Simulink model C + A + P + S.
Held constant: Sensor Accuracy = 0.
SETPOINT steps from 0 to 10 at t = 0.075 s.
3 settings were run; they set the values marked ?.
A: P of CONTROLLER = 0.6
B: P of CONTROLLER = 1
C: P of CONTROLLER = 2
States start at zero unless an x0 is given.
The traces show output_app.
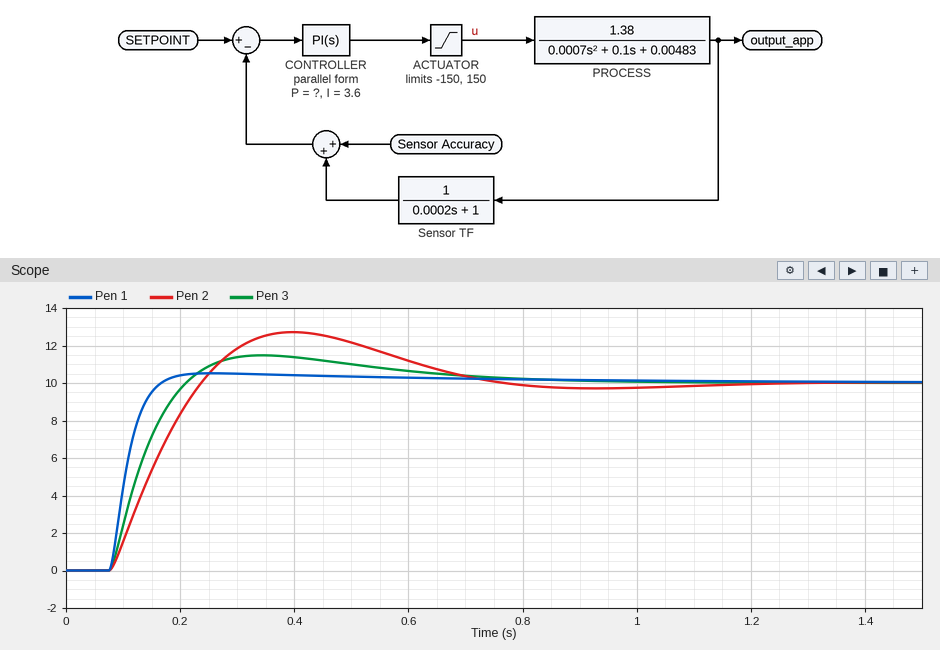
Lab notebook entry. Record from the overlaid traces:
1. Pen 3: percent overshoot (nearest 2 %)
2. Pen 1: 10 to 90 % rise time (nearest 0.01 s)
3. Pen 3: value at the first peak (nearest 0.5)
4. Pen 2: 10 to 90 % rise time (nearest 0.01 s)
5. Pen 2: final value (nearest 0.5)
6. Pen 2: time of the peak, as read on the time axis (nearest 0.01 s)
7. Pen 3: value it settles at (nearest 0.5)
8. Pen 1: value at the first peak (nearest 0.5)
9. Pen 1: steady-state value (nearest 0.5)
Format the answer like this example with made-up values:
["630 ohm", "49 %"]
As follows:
["14 %", "0.06 s", "11.5", "0.12 s", "10.0", "0.40 s", "10.0", "10.5", "10.0"]
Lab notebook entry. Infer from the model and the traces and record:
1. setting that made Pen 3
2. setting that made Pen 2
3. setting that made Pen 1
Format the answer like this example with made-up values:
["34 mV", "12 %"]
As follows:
["B", "A", "C"]
